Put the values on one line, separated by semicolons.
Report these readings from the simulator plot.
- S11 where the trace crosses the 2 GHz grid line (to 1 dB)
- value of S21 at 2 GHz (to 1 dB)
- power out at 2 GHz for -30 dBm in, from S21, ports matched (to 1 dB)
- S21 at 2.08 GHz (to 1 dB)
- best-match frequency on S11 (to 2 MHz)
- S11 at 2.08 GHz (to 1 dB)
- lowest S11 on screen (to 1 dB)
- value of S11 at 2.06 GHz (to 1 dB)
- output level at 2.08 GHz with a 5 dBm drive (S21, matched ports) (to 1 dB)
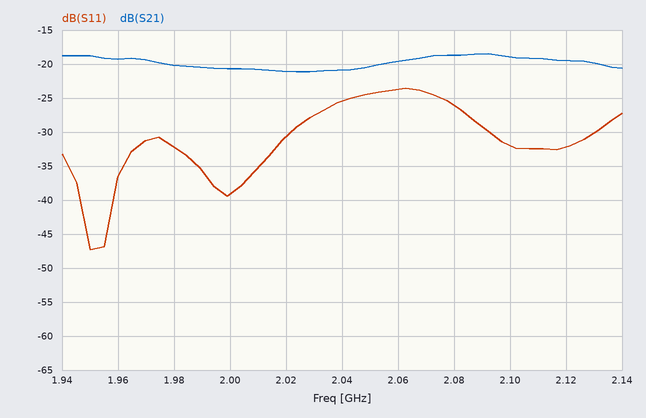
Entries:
-39 dB; -21 dB; -51 dBm; -19 dB; 1.950 GHz; -26 dB; -47 dB; -24 dB; -14 dBm
